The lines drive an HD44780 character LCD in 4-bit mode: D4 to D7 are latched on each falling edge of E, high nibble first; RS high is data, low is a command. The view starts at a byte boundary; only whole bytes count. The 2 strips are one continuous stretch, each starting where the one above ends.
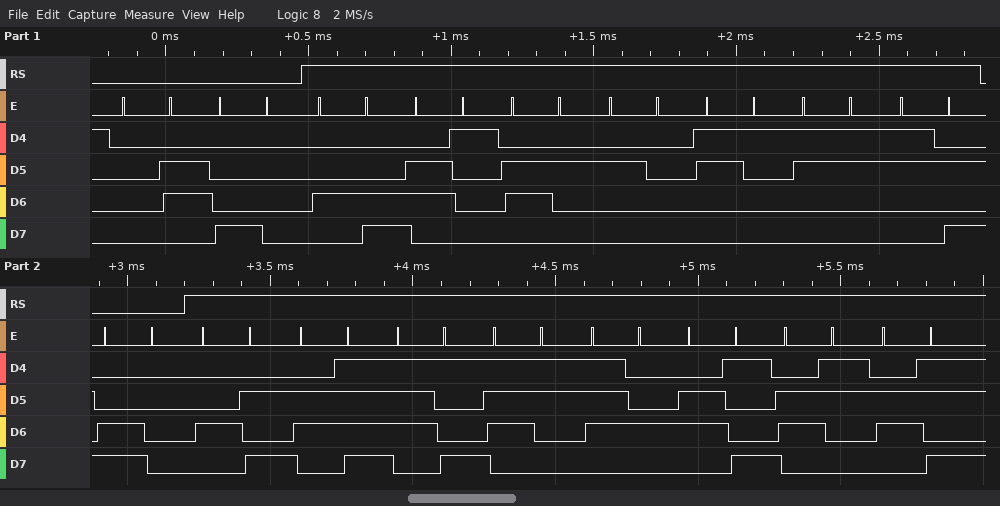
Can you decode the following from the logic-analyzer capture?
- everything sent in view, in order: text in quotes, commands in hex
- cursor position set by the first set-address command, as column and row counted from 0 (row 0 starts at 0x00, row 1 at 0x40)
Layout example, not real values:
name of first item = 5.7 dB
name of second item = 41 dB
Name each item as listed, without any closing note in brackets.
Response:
everything sent in view, in order: text in quotes, commands in hex = 0x06 0x80 "Lab 13:" 0xC0 "Joystick"
cursor position set by the first set-address command, as column and row counted from 0 = column 0, row 0
